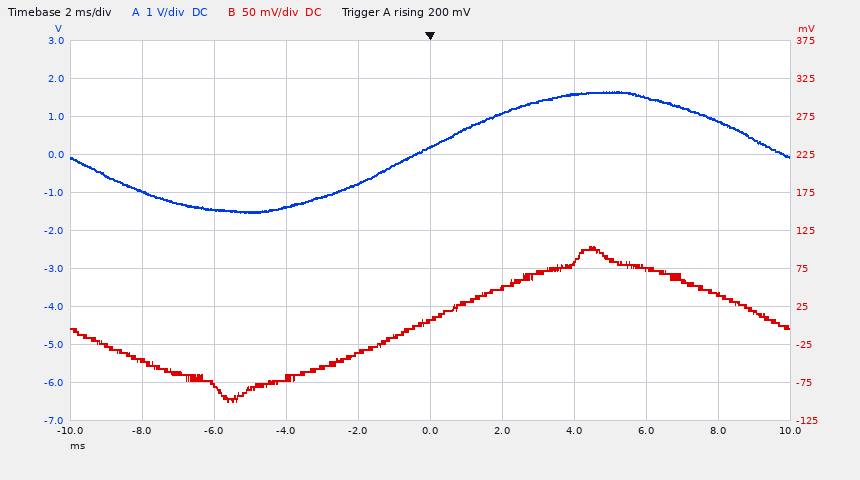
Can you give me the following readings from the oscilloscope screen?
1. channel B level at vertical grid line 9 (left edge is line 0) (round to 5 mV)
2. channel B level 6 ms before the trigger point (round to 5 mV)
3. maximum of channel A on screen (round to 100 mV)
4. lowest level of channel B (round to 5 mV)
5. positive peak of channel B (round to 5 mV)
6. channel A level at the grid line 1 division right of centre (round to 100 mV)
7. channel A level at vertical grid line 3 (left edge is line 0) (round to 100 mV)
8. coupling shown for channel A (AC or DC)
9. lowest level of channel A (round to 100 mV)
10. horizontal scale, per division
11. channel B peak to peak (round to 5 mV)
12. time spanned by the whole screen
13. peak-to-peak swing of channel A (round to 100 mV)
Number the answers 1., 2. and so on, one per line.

1. 40 mV
2. -75 mV
3. 1.7 V
4. -100 mV
5. 105 mV
6. 1.1 V
7. -1.4 V
8. DC
9. -1.5 V
10. 2 ms
11. 205 mV
12. 20 ms
13. 3.2 V
